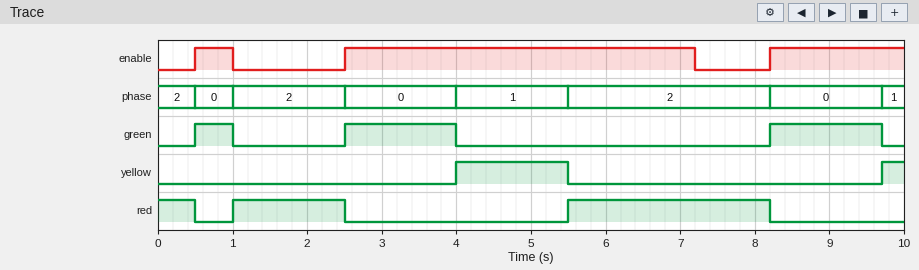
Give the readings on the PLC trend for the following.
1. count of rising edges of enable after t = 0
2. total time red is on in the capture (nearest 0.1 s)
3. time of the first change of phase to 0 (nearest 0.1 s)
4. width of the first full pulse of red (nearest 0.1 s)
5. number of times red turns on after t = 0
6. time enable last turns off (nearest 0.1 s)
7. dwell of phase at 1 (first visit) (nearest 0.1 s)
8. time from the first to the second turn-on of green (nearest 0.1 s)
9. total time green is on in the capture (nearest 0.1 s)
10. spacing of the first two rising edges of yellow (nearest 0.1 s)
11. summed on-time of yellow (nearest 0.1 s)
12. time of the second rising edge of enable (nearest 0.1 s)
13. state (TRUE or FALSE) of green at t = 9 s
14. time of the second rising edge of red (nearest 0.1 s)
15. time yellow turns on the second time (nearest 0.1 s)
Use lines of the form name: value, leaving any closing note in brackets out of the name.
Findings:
count of rising edges of enable after t = 0: 3
total time red is on in the capture: 4.7 s
time of the first change of phase to 0: 0.5 s
width of the first full pulse of red: 1.5 s
number of times red turns on after t = 0: 2
time enable last turns off: 7.2 s
dwell of phase at 1 (first visit): 1.5 s
time from the first to the second turn-on of green: 2.0 s
total time green is on in the capture: 3.5 s
spacing of the first two rising edges of yellow: 5.7 s
summed on-time of yellow: 1.8 s
time of the second rising edge of enable: 2.5 s
state (TRUE or FALSE) of green at t = 9 s: TRUE
time of the second rising edge of red: 5.5 s
time yellow turns on the second time: 9.7 s
